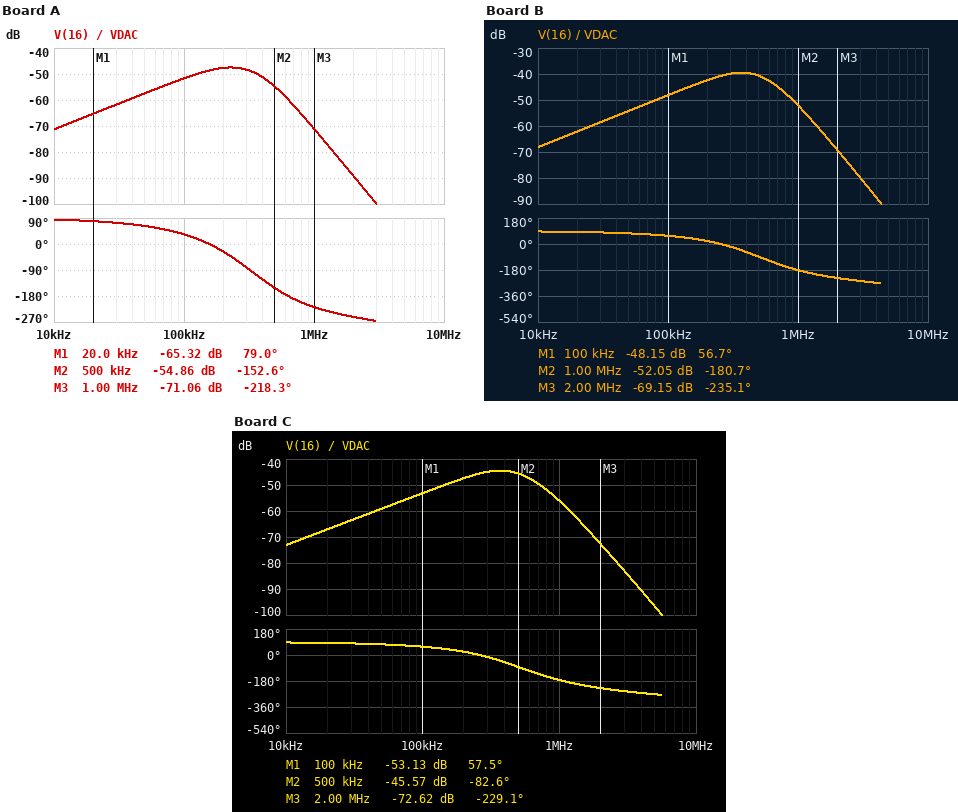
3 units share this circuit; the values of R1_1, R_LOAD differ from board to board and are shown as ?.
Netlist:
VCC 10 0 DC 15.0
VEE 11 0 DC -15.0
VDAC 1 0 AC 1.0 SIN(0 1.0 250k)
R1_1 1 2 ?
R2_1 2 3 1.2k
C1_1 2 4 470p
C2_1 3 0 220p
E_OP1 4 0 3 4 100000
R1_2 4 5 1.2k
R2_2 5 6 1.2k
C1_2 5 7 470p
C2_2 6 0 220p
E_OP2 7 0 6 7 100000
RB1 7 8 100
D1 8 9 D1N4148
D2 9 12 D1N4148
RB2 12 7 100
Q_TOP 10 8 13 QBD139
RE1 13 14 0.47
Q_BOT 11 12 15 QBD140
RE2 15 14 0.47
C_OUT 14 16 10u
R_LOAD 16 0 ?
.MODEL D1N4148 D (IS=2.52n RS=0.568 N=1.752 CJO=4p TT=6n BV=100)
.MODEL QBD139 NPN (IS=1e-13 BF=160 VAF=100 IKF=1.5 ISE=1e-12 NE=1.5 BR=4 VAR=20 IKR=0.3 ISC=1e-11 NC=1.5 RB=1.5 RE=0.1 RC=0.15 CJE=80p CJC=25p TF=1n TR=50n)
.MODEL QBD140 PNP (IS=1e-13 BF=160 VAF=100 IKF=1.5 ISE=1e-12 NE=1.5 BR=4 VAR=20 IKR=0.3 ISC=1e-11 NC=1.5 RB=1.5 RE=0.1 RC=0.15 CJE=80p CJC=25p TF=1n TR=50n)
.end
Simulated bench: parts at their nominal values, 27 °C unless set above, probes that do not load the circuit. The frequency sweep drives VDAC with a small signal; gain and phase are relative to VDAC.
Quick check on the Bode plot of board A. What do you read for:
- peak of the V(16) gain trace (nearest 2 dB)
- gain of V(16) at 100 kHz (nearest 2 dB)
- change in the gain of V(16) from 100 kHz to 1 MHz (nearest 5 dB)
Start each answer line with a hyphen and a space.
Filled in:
- -48 dB
- -52 dB
- -20 dB
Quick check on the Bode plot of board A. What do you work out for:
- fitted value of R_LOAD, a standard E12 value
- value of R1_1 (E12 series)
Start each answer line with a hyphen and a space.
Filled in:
- 27 Ω
- 3.3 kΩ
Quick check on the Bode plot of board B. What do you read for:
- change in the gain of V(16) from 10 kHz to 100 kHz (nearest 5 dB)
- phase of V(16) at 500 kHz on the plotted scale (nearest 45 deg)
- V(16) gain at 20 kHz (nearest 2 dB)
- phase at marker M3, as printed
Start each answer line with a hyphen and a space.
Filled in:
- 20 dB
- -90 deg
- -62 dB
- -235.1 deg
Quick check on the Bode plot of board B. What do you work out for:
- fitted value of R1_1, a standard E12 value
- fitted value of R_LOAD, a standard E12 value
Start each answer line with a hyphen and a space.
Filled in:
- 470 Ω
- 39 Ω
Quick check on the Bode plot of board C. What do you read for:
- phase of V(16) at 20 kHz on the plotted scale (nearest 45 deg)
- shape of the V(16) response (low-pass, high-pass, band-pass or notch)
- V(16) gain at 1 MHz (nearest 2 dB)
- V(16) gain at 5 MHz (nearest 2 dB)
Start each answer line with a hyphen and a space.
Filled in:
- 90 deg
- band-pass
- -56 dB
- -96 dB
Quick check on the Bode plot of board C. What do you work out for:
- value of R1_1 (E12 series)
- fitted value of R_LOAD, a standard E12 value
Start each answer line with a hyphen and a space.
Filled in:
- 390 Ω
- 22 Ω
